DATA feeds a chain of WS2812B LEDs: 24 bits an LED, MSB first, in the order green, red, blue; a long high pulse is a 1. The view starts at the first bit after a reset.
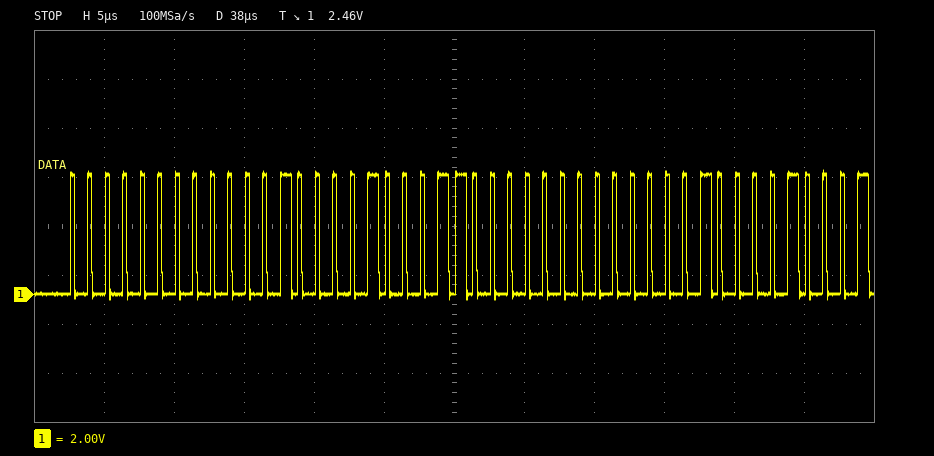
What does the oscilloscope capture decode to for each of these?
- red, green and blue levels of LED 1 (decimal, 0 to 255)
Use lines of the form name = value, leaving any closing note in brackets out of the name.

red, green and blue levels of LED 1 = 8, 0, 70
